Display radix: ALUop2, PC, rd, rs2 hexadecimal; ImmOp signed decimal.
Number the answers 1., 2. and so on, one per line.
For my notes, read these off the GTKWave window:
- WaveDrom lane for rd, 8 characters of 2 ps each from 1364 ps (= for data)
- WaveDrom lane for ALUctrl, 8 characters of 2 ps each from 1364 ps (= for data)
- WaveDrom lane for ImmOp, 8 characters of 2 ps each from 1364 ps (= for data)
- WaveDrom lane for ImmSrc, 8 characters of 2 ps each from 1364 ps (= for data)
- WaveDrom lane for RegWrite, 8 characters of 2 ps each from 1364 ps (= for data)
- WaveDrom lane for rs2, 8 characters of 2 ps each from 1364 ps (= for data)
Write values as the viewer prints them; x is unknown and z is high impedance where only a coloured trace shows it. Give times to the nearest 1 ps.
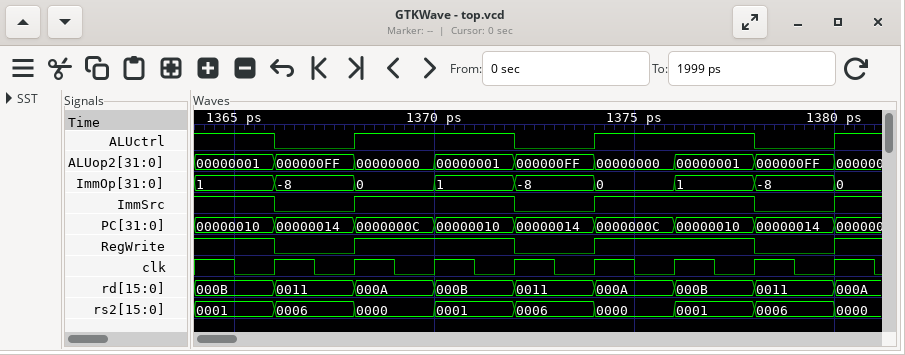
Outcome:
1. {name: 'rd', wave: '========', data: '000B 0011 000A 000B 0011 000A 000B 0011'}
2. {name: 'ALUctrl', wave: '101.01.0'}
3. {name: 'ImmOp', wave: '========', data: '1 -8 0 1 -8 0 1 -8'}
4. {name: 'ImmSrc', wave: '101.01.0'}
5. {name: 'RegWrite', wave: '101.01.0'}
6. {name: 'rs2', wave: '========', data: '0001 0006 0000 0001 0006 0000 0001 0006'}
